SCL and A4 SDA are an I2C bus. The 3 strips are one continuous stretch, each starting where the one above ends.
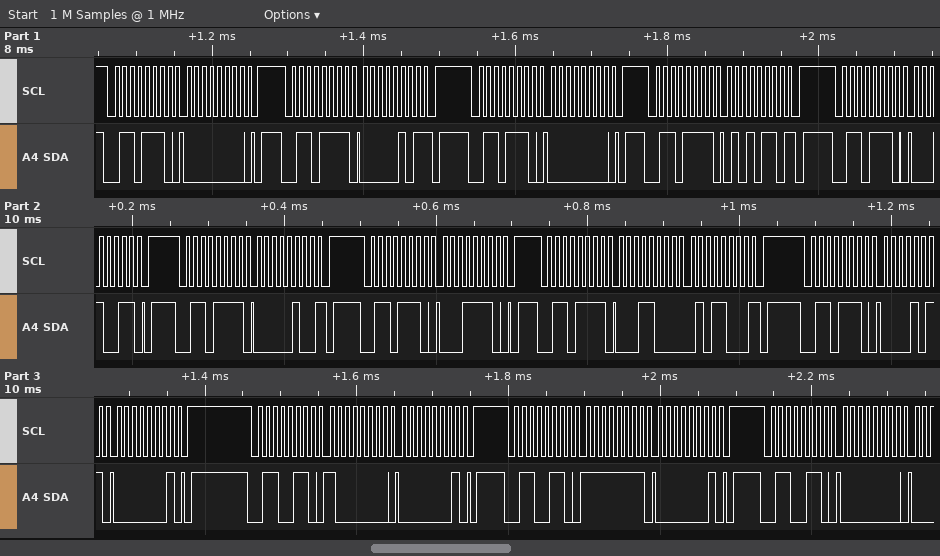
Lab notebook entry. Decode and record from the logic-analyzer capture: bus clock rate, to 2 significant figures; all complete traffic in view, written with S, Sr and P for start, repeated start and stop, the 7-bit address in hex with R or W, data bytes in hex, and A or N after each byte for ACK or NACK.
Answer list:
100 kHz
S 37W A 00 A P S 37R A 05 N P S 37W A 00 A P S 37R A 56 N P S 37W A 13 A P S 37R A 04 N P S 37W A 1E A P S 37R A 18 A 58 N P S 37W A 0B A 01 A P S 33W A 80 A 01 A P S 33W A FF A 01 A P S 33W A 00 A
